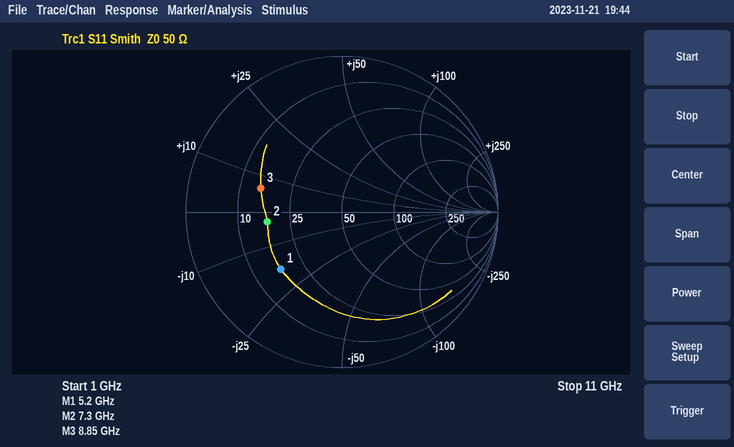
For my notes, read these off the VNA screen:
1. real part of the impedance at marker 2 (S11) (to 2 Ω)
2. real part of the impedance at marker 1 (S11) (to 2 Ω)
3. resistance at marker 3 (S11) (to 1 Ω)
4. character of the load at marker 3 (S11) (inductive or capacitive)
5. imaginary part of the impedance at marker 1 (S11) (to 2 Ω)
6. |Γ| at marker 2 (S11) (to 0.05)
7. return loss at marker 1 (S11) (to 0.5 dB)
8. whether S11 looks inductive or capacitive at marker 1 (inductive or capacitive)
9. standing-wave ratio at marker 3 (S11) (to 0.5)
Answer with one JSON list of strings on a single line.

["18 Ω", "18 Ω", "15 Ω", "inductive", "-18 Ω", "0.50", "5.5 dB", "capacitive", "3.5"]
